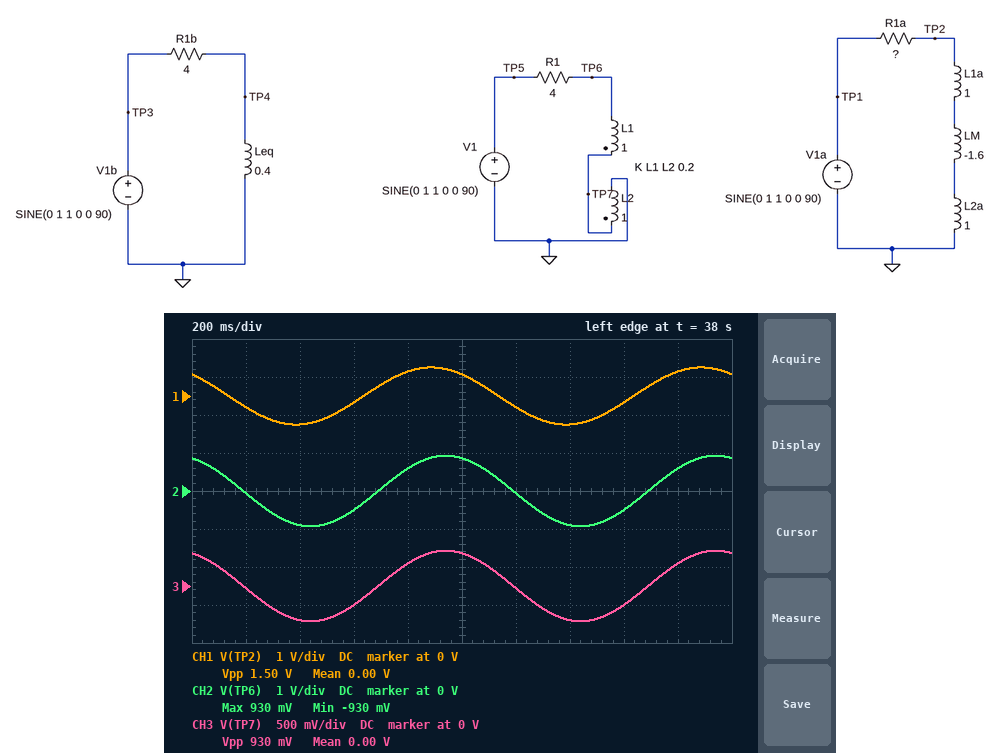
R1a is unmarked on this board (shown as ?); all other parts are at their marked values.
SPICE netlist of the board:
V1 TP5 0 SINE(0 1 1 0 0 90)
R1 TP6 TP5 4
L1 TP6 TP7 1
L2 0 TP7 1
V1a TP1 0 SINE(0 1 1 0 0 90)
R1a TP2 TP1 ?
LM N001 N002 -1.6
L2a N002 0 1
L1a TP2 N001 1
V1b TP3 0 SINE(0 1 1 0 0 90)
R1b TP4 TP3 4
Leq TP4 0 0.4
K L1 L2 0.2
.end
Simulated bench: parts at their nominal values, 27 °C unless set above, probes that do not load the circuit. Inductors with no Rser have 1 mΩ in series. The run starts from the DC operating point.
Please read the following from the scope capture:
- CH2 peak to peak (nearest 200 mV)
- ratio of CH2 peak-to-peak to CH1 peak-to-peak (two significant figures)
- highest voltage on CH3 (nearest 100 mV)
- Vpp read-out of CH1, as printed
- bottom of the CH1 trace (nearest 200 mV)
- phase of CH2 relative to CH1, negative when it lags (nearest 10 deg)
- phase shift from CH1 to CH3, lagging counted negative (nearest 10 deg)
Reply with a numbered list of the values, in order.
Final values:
1. 1.8 V
2. 1.2
3. 500 mV
4. 1.50 V
5. -800 mV
6. -20 deg
7. -20 deg
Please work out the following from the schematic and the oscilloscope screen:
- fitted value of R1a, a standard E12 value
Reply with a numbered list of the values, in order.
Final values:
1. 2.2 Ω
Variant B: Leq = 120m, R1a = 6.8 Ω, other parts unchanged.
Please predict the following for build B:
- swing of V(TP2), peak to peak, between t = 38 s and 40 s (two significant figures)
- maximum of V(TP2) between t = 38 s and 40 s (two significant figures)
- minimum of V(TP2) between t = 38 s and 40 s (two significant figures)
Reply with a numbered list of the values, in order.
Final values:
1. 690 mV
2. 350 mV
3. -350 mV
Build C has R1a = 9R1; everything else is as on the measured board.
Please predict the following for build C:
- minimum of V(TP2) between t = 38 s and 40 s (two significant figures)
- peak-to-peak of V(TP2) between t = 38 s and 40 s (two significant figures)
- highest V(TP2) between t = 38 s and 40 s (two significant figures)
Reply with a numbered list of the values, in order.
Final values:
1. -270 mV
2. 530 mV
3. 270 mV
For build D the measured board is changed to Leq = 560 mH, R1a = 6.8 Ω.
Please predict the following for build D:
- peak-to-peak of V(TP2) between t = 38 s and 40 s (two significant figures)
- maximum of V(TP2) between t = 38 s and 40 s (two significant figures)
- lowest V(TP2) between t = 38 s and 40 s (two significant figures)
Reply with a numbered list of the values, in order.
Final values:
1. 690 mV
2. 350 mV
3. -350 mV
